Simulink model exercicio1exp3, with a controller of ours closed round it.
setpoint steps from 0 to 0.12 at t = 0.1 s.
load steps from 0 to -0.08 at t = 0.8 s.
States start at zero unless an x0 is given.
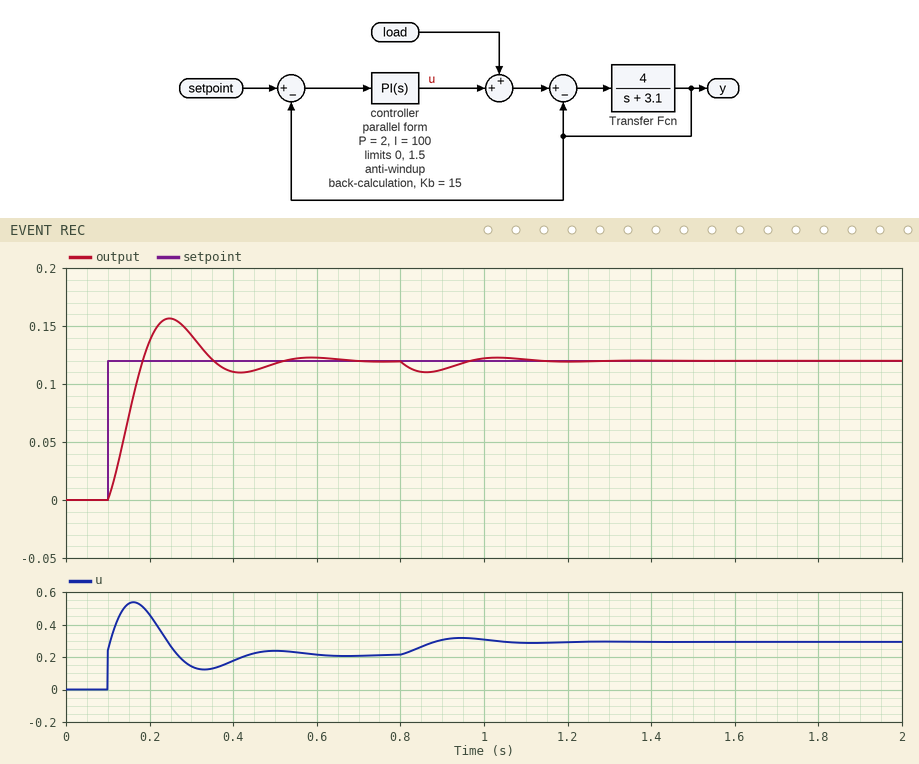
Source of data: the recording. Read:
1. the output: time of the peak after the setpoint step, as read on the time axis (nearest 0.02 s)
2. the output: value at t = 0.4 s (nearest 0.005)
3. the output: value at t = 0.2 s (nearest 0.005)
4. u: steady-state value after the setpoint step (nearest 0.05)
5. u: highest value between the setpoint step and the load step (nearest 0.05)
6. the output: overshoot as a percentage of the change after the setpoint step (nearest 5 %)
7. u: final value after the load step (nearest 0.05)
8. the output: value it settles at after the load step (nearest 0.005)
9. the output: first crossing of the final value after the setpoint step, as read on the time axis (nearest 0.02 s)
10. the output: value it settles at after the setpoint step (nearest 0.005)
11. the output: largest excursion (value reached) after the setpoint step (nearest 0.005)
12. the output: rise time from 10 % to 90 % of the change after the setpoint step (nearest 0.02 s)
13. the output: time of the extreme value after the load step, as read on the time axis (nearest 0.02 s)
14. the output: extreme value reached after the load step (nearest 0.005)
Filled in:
0.24 s
0.110
0.135
0.20
0.55
30 %
0.30
0.120
0.18 s
0.120
0.155
0.06 s
0.86 s
0.110
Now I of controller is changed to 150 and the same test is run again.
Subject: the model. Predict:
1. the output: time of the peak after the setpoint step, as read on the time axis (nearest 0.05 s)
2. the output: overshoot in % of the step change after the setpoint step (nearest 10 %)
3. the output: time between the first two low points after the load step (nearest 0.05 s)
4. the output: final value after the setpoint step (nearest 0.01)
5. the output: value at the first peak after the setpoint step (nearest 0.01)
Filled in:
0.20 s
40 %
0.25 s
0.12
0.17
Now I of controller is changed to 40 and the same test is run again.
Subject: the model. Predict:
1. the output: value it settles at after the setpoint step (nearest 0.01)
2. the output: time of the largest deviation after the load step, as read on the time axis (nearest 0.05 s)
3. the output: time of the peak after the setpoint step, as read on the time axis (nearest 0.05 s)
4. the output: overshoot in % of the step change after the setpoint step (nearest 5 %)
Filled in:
0.12
0.90 s
0.35 s
15 %
